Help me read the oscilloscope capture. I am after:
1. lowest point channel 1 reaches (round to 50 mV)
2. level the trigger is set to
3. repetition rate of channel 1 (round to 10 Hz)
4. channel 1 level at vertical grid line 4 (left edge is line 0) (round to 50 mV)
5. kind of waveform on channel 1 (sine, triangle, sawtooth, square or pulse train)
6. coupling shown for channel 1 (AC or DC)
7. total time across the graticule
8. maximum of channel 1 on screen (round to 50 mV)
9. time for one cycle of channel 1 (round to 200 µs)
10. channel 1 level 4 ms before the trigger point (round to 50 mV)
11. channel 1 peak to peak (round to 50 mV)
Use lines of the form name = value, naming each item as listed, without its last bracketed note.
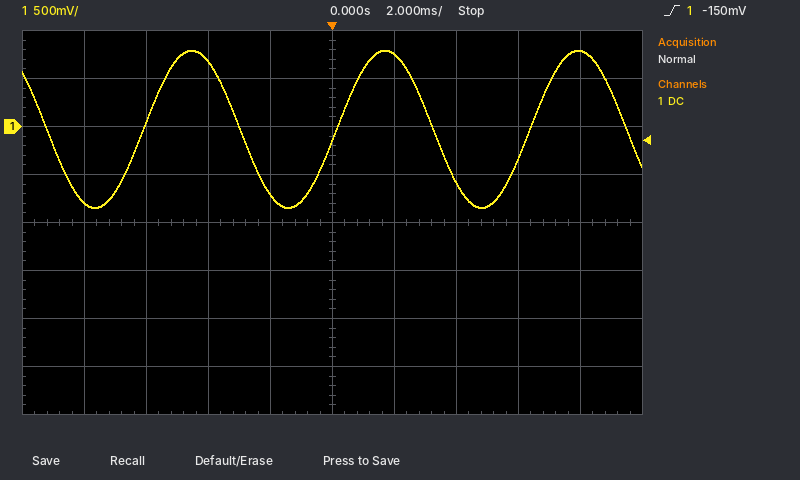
lowest point channel 1 reaches = -850 mV
level the trigger is set to = -150 mV
repetition rate of channel 1 = 160 Hz
channel 1 level at vertical grid line 4 (left edge is line 0) = -700 mV
kind of waveform on channel 1 = sine
coupling shown for channel 1 = DC
total time across the graticule = 20 ms
maximum of channel 1 on screen = 800 mV
time for one cycle of channel 1 = 6.2 ms
channel 1 level 4 ms before the trigger point = 700 mV
channel 1 peak to peak = 1.65 V
